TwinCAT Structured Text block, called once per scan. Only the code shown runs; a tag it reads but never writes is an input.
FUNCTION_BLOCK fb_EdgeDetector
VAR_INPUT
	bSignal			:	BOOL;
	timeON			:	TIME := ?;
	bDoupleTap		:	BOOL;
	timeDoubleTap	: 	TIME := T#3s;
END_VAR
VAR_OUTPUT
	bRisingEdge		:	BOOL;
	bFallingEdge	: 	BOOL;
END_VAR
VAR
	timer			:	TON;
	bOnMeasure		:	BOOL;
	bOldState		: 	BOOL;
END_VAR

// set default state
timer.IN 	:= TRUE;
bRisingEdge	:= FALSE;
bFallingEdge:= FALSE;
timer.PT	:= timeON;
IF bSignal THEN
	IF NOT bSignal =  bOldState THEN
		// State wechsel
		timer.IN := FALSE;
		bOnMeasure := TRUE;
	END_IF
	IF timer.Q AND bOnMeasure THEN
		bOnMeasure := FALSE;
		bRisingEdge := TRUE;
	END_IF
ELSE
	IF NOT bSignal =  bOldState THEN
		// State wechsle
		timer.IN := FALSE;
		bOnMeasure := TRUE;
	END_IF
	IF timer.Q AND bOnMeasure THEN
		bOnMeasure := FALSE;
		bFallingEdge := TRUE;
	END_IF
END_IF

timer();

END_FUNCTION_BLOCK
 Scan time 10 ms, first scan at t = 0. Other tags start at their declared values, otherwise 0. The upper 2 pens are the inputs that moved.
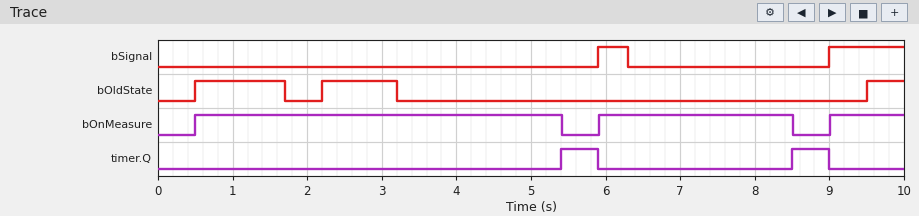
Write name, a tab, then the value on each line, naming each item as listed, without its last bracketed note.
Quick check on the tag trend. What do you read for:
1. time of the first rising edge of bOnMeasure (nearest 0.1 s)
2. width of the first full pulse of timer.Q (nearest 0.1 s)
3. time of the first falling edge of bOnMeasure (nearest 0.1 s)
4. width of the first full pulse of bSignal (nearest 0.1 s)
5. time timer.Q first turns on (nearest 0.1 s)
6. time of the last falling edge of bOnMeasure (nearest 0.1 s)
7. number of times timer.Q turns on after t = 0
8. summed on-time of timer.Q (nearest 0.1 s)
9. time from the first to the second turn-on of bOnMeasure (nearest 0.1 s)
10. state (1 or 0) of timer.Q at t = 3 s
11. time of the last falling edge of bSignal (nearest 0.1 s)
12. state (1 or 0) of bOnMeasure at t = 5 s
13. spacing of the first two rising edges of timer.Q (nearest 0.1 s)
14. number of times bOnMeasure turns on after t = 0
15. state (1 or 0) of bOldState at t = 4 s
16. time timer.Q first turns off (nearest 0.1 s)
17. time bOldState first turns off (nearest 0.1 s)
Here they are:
time of the first rising edge of bOnMeasure	0.5 s
width of the first full pulse of timer.Q	0.5 s
time of the first falling edge of bOnMeasure	5.4 s
width of the first full pulse of bSignal	0.4 s
time timer.Q first turns on	5.4 s
time of the last falling edge of bOnMeasure	8.5 s
number of times timer.Q turns on after t = 0	2
summed on-time of timer.Q	1.0 s
time from the first to the second turn-on of bOnMeasure	5.4 s
state (1 or 0) of timer.Q at t = 3 s	0
time of the last falling edge of bSignal	6.3 s
state (1 or 0) of bOnMeasure at t = 5 s	1
spacing of the first two rising edges of timer.Q	3.1 s
number of times bOnMeasure turns on after t = 0	3
state (1 or 0) of bOldState at t = 4 s	0
time timer.Q first turns off	5.9 s
time bOldState first turns off	1.7 s
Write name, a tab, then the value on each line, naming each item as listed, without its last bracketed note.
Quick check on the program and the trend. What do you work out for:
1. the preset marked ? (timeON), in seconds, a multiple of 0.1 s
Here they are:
the preset marked ? (timeON), in seconds, a multiple of 0.1 s	2.2 s
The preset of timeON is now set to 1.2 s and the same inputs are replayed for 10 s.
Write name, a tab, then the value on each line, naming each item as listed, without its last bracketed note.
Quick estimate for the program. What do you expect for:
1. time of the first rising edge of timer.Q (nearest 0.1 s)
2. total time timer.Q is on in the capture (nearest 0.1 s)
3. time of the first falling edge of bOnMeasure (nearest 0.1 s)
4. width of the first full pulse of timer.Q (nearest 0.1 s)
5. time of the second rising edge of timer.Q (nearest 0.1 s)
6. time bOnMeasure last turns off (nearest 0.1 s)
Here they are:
time of the first rising edge of timer.Q	4.4 s
total time timer.Q is on in the capture	3.0 s
time of the first falling edge of bOnMeasure	4.4 s
width of the first full pulse of timer.Q	1.5 s
time of the second rising edge of timer.Q	7.5 s
time bOnMeasure last turns off	7.5 s
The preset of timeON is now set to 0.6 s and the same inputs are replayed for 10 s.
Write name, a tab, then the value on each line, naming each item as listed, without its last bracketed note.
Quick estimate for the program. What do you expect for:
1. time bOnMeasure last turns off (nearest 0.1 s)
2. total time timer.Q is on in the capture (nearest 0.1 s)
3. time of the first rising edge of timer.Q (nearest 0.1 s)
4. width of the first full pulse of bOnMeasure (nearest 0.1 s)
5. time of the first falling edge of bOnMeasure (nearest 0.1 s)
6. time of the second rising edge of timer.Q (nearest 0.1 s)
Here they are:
time bOnMeasure last turns off	6.9 s
total time timer.Q is on in the capture	4.2 s
time of the first rising edge of timer.Q	3.8 s
width of the first full pulse of bOnMeasure	3.3 s
time of the first falling edge of bOnMeasure	3.8 s
time of the second rising edge of timer.Q	6.9 s
